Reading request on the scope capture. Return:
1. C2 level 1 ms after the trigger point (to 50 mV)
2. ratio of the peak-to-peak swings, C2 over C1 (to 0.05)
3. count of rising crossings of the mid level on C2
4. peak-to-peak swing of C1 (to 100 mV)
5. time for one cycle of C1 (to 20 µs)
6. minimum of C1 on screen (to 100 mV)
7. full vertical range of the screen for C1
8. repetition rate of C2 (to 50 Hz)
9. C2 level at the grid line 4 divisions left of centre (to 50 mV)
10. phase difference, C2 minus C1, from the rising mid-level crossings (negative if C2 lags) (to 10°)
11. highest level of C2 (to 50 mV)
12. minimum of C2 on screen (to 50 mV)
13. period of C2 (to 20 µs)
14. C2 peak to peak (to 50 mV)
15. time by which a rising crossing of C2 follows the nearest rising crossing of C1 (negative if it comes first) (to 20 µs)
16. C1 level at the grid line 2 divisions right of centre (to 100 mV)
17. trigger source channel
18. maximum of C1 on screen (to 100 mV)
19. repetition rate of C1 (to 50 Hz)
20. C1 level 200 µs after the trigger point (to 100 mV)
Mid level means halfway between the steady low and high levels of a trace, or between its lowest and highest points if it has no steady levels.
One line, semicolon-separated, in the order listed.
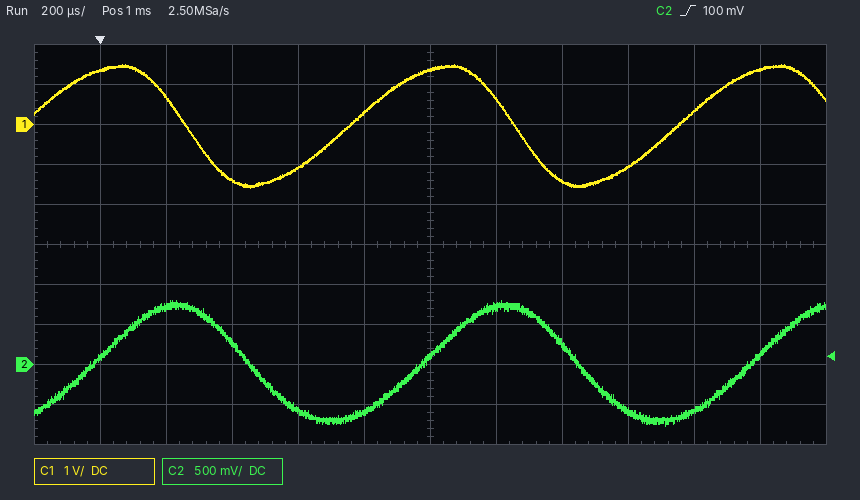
100 mV; 0.50; 3; 3.1 V; 1.00 ms; -1.6 V; 10 V; 1.00 kHz; 700 mV; -80°; 800 mV; -750 mV; 1.00 ms; 1.55 V; +220 µs; -1.4 V; C2; 1.5 V; 1.00 kHz; 700 mV
